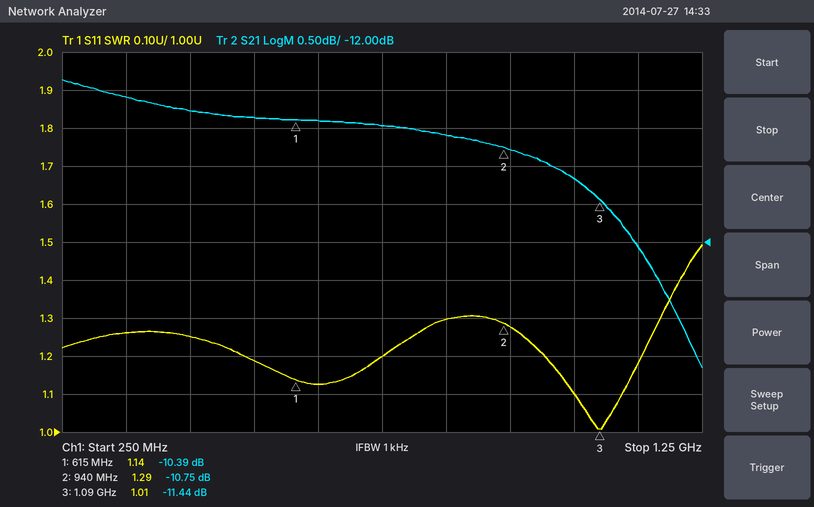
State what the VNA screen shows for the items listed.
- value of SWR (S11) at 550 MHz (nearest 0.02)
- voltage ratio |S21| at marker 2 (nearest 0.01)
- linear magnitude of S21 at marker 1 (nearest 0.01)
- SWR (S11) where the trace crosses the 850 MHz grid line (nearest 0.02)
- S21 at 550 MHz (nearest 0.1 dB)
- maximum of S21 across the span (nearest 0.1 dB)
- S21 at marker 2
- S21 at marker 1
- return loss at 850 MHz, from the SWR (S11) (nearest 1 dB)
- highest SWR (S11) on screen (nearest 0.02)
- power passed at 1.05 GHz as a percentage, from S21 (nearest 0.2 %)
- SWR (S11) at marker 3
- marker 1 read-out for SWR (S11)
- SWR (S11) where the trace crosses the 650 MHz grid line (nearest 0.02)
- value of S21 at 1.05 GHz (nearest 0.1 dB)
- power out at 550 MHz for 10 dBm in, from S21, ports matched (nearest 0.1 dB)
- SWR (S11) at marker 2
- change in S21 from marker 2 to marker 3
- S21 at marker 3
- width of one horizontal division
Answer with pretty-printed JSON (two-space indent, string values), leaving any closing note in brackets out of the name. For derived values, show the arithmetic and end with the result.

{
  "value of SWR (S11) at 550 MHz": "1.18",
  "voltage ratio |S21| at marker 2": "10^(-10.75/20) ≈ 0.29",
  "linear magnitude of S21 at marker 1": "10^(-10.39/20) ≈ 0.30",
  "SWR (S11) where the trace crosses the 850 MHz grid line": "1.30",
  "S21 at 550 MHz": "-10.4 dB",
  "maximum of S21 across the span": "-9.9 dB",
  "S21 at marker 2": "-10.75 dB",
  "S21 at marker 1": "-10.39 dB",
  "return loss at 850 MHz, from the SWR (S11)": "−20 log10((1.3 − 1)/(1.3 + 1)) ≈ 18 dB",
  "highest SWR (S11) on screen": "1.50",
  "power passed at 1.05 GHz as a percentage, from S21": "10^(-11.2/10) ≈ 7.6 %",
  "SWR (S11) at marker 3": "1.01",
  "marker 1 read-out for SWR": "1.14",
  "SWR (S11) where the trace crosses the 650 MHz grid line": "1.12",
  "value of S21 at 1.05 GHz": "-11.2 dB",
  "power out at 550 MHz for 10 dBm in, from S21, ports matched": "10 dBm + (-10.4 dB) = -0.4 dBm",
  "SWR (S11) at marker 2": "1.29",
  "change in S21 from marker 2 to marker 3": "-11.44 − (-10.75) = -0.69 dB",
  "S21 at marker 3": "-11.44 dB",
  "width of one horizontal division": "100 MHz"
}
